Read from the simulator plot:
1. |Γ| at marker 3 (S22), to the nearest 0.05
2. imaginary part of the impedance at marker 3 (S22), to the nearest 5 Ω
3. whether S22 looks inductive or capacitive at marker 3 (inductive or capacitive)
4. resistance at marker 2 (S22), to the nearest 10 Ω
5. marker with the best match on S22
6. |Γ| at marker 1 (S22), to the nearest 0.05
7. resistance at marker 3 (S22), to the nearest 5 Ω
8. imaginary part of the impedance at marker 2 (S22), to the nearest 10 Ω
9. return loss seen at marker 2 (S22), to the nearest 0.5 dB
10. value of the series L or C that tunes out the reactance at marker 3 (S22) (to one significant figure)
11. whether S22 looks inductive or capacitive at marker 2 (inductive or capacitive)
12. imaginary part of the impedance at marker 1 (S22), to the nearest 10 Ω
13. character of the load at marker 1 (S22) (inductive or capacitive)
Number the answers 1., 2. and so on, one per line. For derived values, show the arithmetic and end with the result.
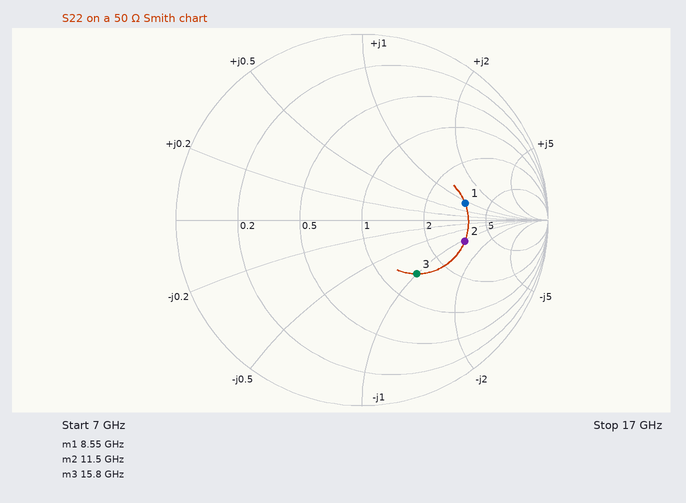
1. 0.40
2. -50 Ω
3. capacitive
4. 160 Ω
5. marker 3
6. 0.55
7. 70 Ω
8. -50 Ω
9. 5.0 dB
10. L = 50 Ω/(2π × 15.8 GHz) ≈ 504 pH, so 500 pH to one significant figure
11. capacitive
12. +40 Ω
13. inductive
